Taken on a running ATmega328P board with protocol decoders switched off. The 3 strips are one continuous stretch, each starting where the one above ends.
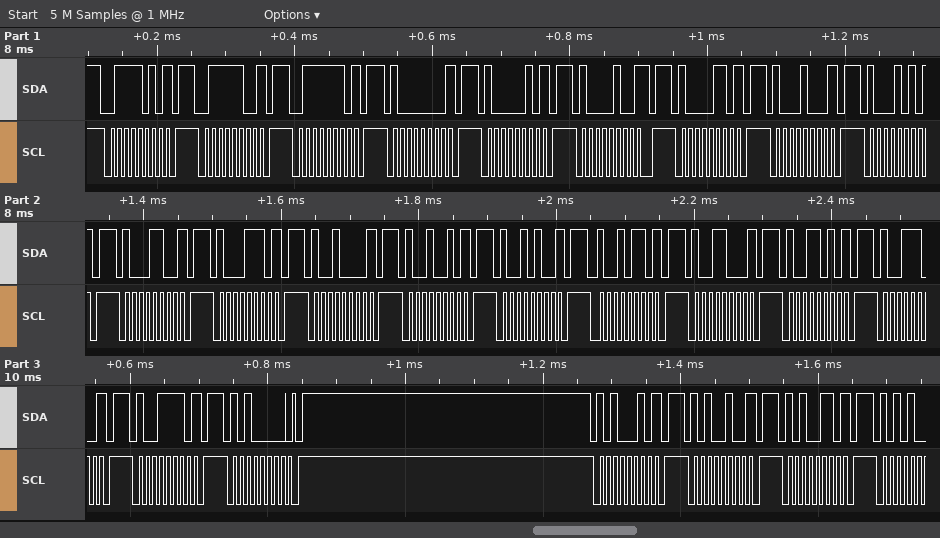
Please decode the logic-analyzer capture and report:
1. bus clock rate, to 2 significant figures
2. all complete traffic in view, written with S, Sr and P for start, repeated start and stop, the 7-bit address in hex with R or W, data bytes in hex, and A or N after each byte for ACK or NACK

100 kHz
S 3DW N P S 3EW N P S 3FW N P S 40W N P S 41W N P S 42W N P S 43W N P S 44W N P S 45W N P S 46W N P S 47W N P S 48W N P S 49W N P S 4AW N P S 4BW N P S 4CW N P S 4DW N P S 4EW N P S 4FW N P S 50W A P S 51W N P S 52W N P S 53W N P
